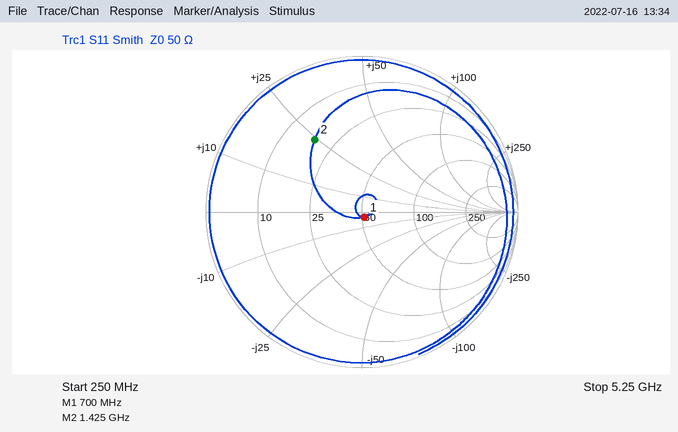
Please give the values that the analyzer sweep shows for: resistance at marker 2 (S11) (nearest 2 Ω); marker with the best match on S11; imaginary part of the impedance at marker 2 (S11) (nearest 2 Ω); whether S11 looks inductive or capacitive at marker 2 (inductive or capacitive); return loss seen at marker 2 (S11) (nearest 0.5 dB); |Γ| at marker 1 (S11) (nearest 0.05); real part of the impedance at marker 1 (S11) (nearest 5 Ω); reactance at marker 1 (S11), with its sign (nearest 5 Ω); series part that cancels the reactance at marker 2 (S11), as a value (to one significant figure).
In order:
18 Ω
marker 1
+24 Ω
inductive
5.0 dB
0.05
50 Ω
-5 Ω
5 pF
